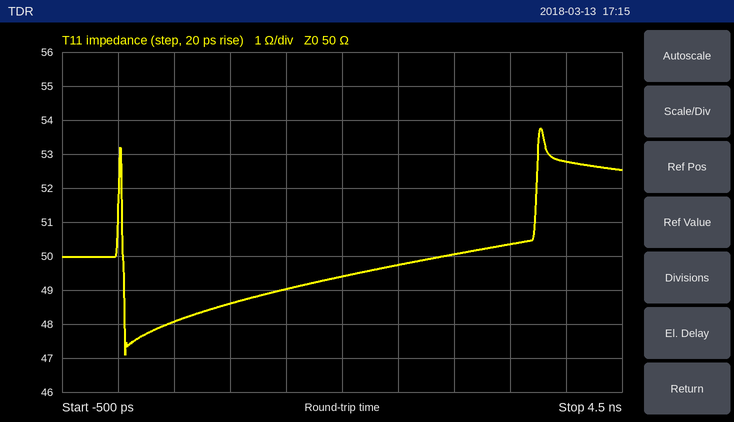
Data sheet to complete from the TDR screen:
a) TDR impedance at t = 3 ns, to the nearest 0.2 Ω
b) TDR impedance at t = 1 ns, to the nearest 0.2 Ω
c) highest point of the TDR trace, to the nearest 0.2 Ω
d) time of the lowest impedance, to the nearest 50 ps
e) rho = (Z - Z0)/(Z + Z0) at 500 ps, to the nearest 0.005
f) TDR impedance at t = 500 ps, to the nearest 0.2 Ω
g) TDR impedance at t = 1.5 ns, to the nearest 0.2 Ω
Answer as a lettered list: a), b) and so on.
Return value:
a) 50.0 Ω
b) 48.6 Ω
c) 53.8 Ω
d) 50 ps
e) -0.020
f) 48.0 Ω
g) 49.0 Ω
